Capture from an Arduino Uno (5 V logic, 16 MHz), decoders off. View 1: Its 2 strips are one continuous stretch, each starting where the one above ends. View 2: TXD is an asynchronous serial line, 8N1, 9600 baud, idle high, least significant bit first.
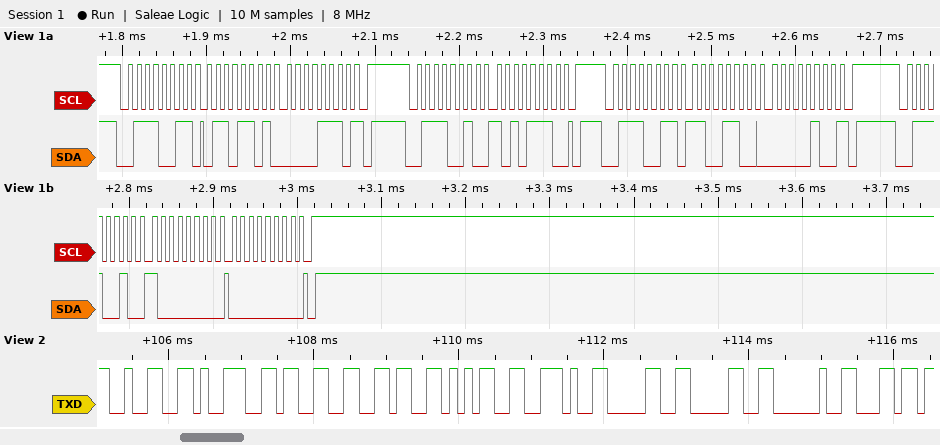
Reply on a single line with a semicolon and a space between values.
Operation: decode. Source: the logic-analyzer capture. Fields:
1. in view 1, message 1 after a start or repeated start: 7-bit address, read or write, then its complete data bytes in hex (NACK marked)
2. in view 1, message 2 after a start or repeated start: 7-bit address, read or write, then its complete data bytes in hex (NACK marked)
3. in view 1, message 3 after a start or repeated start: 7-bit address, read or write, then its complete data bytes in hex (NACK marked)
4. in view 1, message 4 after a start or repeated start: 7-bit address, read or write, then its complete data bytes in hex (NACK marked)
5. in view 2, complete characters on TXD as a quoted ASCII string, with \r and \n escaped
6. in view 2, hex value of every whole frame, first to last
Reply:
0x39 read: 6D 0E NACK; 0x39 write: AE; 0x39 read: CC 04 NACK; 0x39 write: 80 00; "29365.00 l"; 0x32 0x39 0x33 0x36 0x35 0x2E 0x30 0x30 0x20 0x6C
